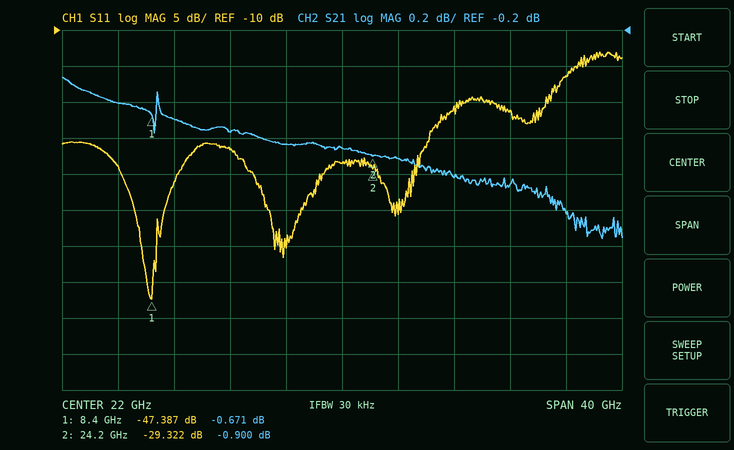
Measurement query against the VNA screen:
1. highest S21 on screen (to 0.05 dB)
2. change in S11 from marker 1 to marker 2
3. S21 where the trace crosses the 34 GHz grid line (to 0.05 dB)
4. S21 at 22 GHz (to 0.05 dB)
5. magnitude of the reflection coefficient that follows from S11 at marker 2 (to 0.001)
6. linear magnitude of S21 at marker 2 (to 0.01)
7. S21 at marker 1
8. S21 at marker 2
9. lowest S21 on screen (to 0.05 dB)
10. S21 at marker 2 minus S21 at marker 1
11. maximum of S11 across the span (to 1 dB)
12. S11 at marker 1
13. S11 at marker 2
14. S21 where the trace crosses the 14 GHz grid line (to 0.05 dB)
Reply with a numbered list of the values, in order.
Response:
1. -0.45 dB
2. 18.065 dB
3. -1.05 dB
4. -0.85 dB
5. 0.034
6. 0.90
7. -0.671 dB
8. -0.900 dB
9. -1.35 dB
10. -0.229 dB
11. -13 dB
12. -47.387 dB
13. -29.322 dB
14. -0.75 dB
